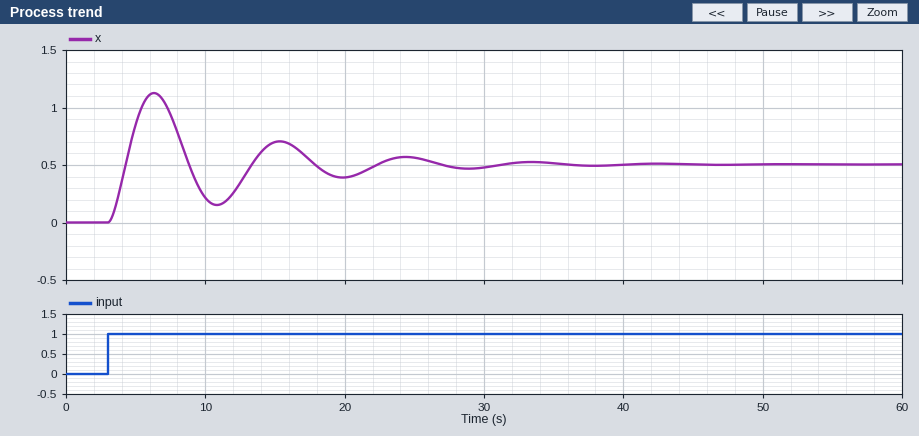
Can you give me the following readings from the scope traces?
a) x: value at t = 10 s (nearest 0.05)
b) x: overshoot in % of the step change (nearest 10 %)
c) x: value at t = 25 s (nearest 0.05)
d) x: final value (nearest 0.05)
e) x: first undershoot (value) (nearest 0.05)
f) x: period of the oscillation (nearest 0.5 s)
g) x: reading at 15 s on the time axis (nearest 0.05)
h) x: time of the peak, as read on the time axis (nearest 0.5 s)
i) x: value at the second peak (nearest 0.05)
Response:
0.20
120 %
0.55
0.50
0.15
9.0 s
0.70
6.5 s
0.70
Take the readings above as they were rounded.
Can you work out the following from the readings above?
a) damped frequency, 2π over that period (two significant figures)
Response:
0.70 rad/s
